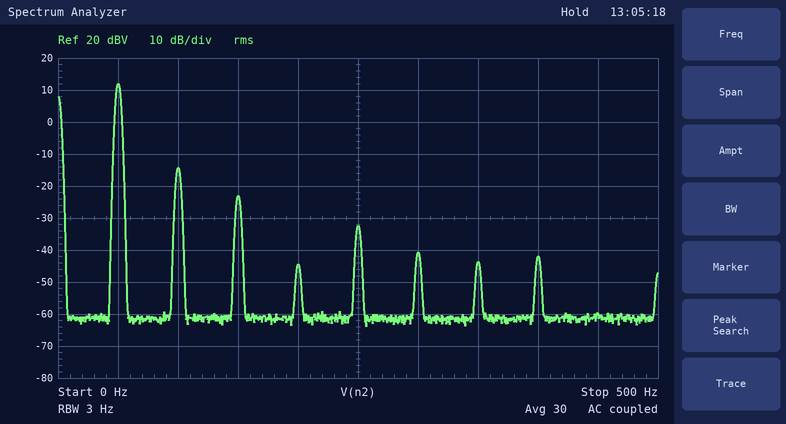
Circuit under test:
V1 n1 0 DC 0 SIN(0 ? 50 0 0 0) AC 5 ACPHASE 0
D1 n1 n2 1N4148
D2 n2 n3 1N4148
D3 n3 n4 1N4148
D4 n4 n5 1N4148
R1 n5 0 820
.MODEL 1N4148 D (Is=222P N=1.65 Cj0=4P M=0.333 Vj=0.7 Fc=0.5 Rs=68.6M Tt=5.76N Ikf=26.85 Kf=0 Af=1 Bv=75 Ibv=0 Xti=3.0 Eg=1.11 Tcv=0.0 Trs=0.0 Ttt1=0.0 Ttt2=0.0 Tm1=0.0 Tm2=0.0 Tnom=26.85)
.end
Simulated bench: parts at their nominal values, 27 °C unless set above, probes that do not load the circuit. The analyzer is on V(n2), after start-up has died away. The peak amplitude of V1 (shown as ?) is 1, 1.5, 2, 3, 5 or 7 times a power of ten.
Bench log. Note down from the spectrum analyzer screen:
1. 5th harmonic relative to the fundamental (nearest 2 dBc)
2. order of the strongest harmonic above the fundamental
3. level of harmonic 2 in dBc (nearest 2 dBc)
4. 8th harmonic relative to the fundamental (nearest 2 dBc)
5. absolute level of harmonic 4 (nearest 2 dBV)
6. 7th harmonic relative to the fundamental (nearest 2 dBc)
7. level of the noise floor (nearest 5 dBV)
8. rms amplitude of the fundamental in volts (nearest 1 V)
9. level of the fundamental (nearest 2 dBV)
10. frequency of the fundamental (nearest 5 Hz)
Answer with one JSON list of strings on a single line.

["-44 dBc", "2", "-26 dBc", "-54 dBc", "-44 dBV", "-56 dBc", "-60 dBV", "4 V", "12 dBV", "50 Hz"]
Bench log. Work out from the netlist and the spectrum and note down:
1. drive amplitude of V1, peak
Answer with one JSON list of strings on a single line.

["7 V"]
